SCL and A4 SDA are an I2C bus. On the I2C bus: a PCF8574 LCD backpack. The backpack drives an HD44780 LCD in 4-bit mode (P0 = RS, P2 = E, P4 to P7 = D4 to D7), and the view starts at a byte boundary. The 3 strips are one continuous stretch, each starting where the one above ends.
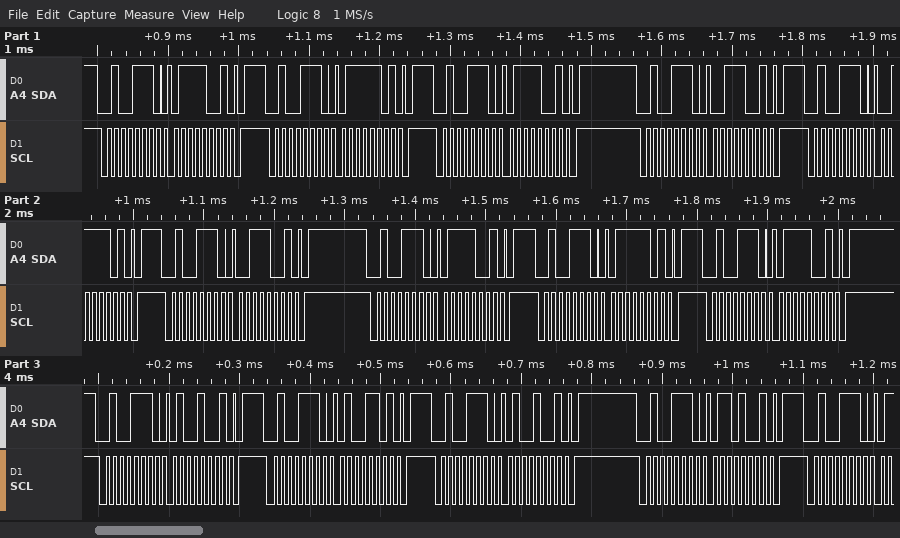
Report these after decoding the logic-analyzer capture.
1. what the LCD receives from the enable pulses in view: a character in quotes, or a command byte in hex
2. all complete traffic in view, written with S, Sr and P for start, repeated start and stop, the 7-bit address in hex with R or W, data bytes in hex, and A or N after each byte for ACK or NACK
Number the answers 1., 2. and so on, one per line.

1. 's' 't'
2. S 27W A 79 A P S 27W A 7D A P S 27W A 79 A P S 27W A 39 A P S 27W A 3D A P S 27W A 39 A P S 27W A 79 A P S 27W A 7D A P S 27W A 79 A P S 27W A 49 A P S 27W A 4D A P S 27W A 49 A P S 27W A 69 A P S 27W A
